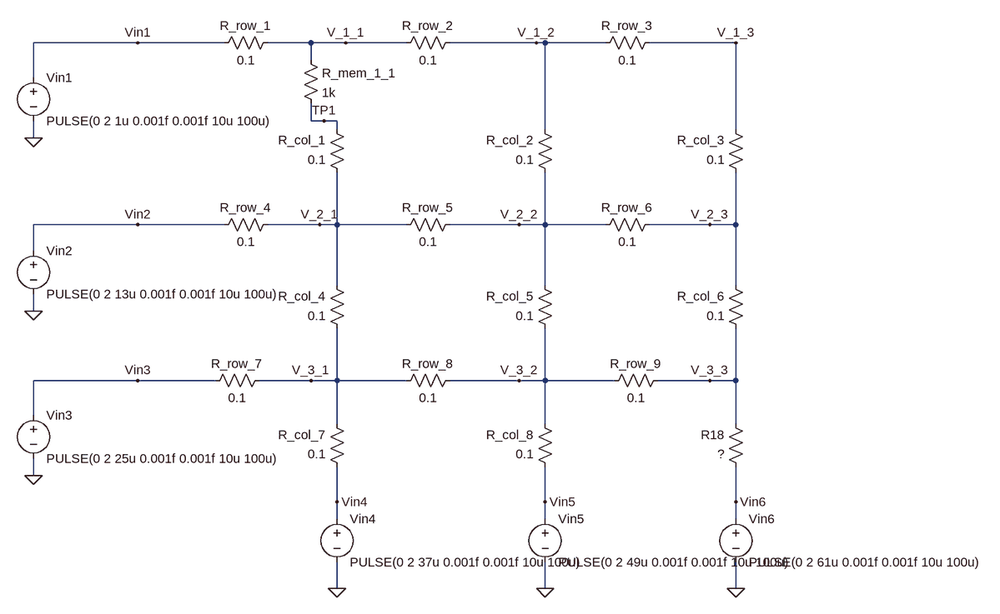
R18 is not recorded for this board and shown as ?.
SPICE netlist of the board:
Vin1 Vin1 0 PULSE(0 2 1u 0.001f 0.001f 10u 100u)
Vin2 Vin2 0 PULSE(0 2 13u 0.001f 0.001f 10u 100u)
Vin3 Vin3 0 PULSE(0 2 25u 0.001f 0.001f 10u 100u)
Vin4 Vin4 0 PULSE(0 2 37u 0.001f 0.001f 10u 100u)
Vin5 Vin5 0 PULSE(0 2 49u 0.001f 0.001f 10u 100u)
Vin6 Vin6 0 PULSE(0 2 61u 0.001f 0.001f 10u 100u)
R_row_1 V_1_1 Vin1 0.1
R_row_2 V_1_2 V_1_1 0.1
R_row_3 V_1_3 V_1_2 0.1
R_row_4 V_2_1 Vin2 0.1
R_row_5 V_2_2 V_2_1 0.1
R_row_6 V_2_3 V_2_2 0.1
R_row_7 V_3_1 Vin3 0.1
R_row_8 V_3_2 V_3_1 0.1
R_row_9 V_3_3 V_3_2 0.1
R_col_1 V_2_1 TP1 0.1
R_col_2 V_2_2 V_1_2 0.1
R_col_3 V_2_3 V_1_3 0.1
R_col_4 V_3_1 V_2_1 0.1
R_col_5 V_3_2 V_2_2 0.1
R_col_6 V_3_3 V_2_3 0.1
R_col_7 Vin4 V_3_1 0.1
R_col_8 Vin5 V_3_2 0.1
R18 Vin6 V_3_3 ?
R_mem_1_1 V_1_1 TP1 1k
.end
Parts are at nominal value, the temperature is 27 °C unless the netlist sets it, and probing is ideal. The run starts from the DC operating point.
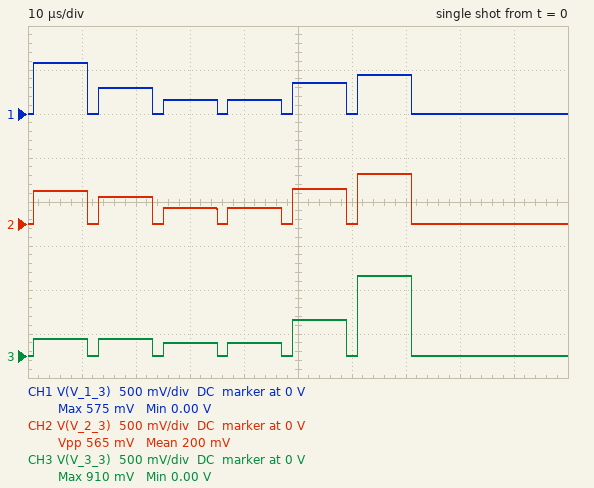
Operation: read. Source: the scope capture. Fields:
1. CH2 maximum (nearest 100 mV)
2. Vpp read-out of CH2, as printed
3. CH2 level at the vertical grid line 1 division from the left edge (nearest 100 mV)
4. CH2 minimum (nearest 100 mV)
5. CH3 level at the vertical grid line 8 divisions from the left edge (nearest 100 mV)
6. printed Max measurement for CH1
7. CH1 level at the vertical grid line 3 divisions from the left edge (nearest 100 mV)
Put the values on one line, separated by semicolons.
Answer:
600 mV; 565 mV; 400 mV; 0 V; 0 V; 575 mV; 200 mV
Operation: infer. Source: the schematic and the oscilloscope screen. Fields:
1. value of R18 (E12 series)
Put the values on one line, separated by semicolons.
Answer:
0.12 Ω
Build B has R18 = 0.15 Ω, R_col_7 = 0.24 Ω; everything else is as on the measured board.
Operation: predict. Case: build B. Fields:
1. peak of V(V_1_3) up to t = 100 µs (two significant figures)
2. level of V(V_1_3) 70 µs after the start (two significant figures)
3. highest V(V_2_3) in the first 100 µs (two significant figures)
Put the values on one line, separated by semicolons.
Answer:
590 mV; 390 mV; 500 mV
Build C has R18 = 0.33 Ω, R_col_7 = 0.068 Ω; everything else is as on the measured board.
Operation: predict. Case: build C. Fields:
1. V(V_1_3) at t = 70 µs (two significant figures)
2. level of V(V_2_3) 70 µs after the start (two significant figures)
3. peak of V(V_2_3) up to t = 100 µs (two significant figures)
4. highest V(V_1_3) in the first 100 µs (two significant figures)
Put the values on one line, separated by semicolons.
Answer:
220 mV; 290 mV; 490 mV; 610 mV
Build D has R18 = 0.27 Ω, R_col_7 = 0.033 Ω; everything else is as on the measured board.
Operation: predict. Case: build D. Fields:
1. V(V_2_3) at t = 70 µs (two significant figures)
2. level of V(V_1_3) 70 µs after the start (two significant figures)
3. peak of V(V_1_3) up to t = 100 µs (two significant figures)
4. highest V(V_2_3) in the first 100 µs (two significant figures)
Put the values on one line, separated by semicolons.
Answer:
330 mV; 250 mV; 600 mV; 450 mV
